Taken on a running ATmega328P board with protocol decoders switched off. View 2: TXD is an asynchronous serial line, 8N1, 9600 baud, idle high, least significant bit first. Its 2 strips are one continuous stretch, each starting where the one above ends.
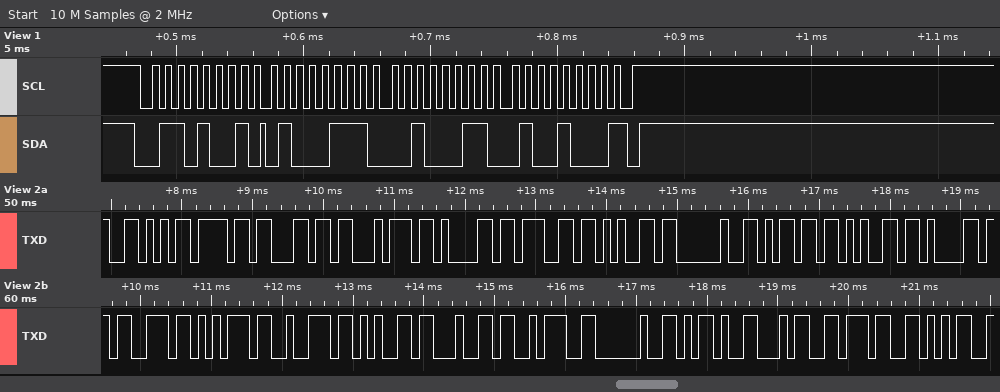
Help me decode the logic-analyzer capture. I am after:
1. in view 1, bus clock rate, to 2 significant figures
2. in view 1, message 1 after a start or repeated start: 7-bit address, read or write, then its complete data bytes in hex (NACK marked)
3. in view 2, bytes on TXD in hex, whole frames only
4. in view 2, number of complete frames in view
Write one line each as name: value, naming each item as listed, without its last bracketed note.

in view 1, bus clock rate, to 2 significant figures: 100 kHz
in view 1, message 1 after a start or repeated start: 7-bit address, read or write, then its complete data bytes in hex: 0x34 read: 47 23 48 NACK
in view 2, bytes on TXD in hex, whole frames only: 56 6F 6C 74 61 67 65 20 6D 65 61 73 75 72 65 64 3A 20 2D 34 37 35
in view 2, number of complete frames in view: 22
